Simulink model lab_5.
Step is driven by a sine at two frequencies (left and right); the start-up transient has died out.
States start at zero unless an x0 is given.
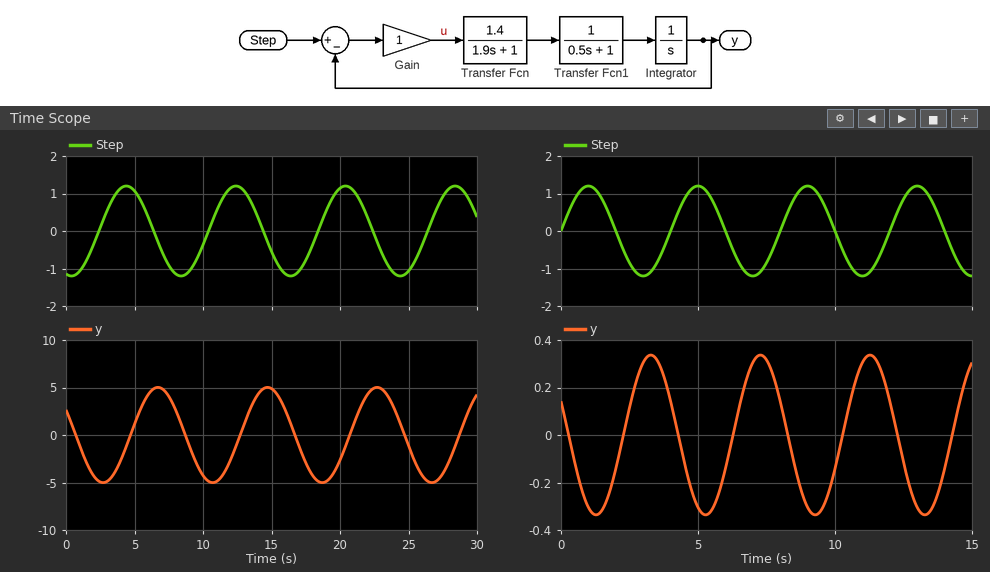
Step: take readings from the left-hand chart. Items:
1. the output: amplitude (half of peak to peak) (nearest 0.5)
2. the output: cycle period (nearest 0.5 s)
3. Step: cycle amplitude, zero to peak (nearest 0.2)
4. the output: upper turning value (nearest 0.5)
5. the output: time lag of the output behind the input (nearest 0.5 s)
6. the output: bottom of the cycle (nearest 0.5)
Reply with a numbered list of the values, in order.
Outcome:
1. 5.0
2. 8.0 s
3. 1.2
4. 5.0
5. 2.5 s
6. -5.0
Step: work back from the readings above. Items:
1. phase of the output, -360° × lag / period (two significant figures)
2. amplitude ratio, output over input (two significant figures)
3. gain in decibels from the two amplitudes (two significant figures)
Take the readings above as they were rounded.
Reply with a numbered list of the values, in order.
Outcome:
1. -110°
2. 4.2
3. 12 dB
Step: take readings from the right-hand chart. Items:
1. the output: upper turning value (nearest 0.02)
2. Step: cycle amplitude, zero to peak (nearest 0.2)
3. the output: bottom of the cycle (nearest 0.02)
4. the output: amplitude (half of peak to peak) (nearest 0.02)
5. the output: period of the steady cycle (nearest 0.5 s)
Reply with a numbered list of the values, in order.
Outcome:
1. 0.34
2. 1.2
3. -0.34
4. 0.34
5. 4.0 s
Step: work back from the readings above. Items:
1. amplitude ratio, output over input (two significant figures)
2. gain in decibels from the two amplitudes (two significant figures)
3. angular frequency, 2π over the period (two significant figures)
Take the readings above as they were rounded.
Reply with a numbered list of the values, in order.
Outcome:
1. 0.28
2. -11 dB
3. 1.6 rad/s
